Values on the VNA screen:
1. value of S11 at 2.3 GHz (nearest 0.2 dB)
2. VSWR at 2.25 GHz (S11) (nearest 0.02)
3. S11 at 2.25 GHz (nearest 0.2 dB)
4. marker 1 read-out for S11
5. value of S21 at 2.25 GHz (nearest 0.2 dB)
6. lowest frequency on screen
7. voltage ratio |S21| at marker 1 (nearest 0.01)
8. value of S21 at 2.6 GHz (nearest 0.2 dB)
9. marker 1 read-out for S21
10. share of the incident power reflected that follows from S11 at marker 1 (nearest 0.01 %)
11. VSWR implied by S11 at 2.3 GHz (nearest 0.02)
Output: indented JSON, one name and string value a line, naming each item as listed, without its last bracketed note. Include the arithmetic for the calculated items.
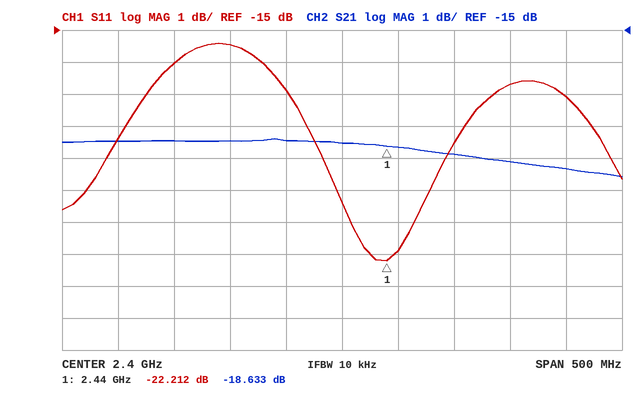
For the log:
{
  "value of S11 at 2.3 GHz": "-15.4 dB",
  "VSWR at 2.25 GHz (S11)": "|Γ| = 10^(-16/20) = 0.1585; VSWR = (1 + 0.1585)/(1 − 0.1585) ≈ 1.38",
  "S11 at 2.25 GHz": "-16.0 dB",
  "marker 1 read-out for S11": "-22.212 dB",
  "value of S21 at 2.25 GHz": "-18.4 dB",
  "lowest frequency on screen": "2.15 GHz",
  "voltage ratio |S21| at marker 1": "10^(-18.633/20) ≈ 0.12",
  "value of S21 at 2.6 GHz": "-19.4 dB",
  "marker 1 read-out for S21": "-18.633 dB",
  "share of the incident power reflected that follows from S11 at marker 1": "10^(-22.212/10) ≈ 0.60 %",
  "VSWR implied by S11 at 2.3 GHz": "|Γ| = 10^(-15.4/20) = 0.1698; VSWR = (1 + 0.1698)/(1 − 0.1698) ≈ 1.41, so 1.40 to the nearest 0.02"
}
